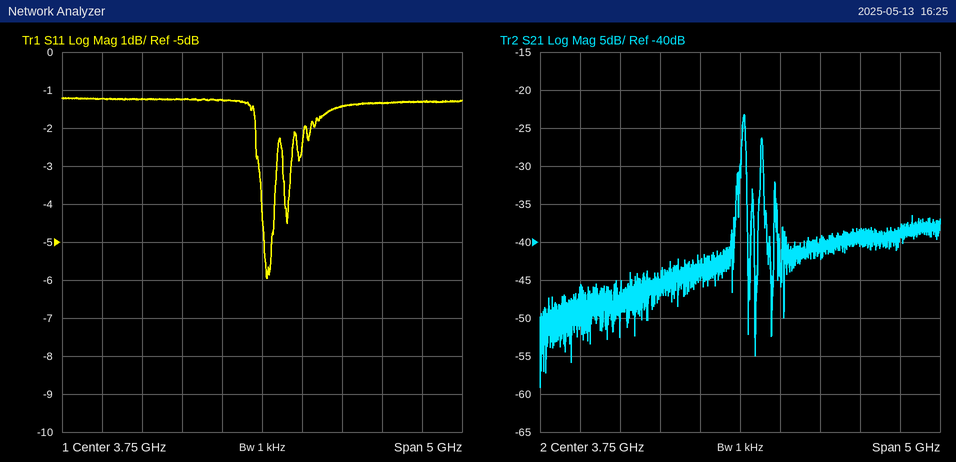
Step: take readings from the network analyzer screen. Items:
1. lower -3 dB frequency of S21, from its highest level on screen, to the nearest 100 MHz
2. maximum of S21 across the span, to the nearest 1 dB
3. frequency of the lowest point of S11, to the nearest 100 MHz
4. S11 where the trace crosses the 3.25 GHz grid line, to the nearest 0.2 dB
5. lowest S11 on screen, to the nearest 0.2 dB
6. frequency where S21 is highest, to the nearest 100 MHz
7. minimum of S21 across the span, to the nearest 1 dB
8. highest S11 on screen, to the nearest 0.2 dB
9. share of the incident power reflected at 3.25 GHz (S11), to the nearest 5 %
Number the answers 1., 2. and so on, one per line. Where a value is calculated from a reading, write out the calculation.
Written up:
1. 3.8 GHz
2. -23 dB
3. 3.8 GHz
4. -1.2 dB
5. -6.0 dB
6. 3.8 GHz
7. -59 dB
8. -1.2 dB
9. 10^(-1.2/10) ≈ 75.9 %, so 75 % to the nearest 5 %
